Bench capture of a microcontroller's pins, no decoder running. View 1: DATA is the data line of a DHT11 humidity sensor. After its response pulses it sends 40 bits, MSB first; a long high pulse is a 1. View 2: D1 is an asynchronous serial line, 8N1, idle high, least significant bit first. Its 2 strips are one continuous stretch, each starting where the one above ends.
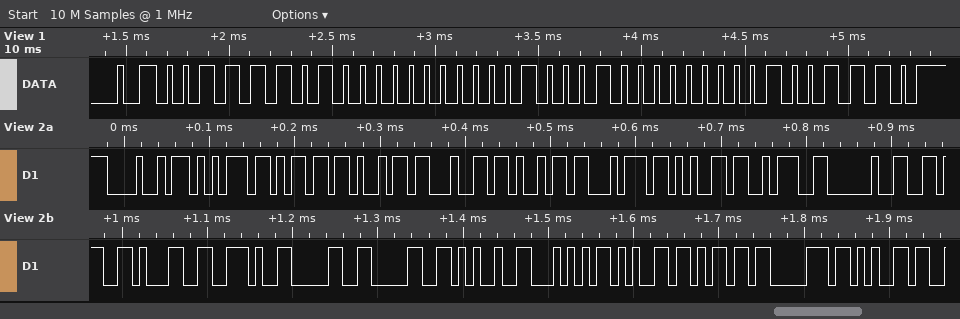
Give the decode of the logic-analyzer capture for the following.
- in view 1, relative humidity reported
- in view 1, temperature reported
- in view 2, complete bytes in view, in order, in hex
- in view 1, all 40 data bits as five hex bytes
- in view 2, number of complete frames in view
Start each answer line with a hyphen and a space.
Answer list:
- 61 %
- 17.0 °C
- 0x48 0x75 0x6D 0x69 0x64 0x69 0x74 0x65 0x3A 0x20 0x36 0x31 0x2E 0x30 0x30 0x25 0x54 0x65 0x6D 0x70 0x65
- 3D 00 11 00 4E
- 21
